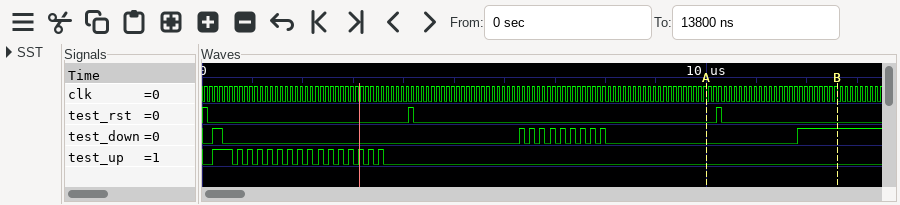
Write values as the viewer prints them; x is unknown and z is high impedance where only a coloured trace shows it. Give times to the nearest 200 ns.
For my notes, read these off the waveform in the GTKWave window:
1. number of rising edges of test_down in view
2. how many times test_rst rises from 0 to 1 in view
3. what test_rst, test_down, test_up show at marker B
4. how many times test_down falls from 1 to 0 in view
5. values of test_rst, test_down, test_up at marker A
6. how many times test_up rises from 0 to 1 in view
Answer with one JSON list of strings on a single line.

["11", "2", "test_rst=0, test_down=1, test_up=0", "10", "test_rst=0, test_down=0, test_up=0", "16"]
